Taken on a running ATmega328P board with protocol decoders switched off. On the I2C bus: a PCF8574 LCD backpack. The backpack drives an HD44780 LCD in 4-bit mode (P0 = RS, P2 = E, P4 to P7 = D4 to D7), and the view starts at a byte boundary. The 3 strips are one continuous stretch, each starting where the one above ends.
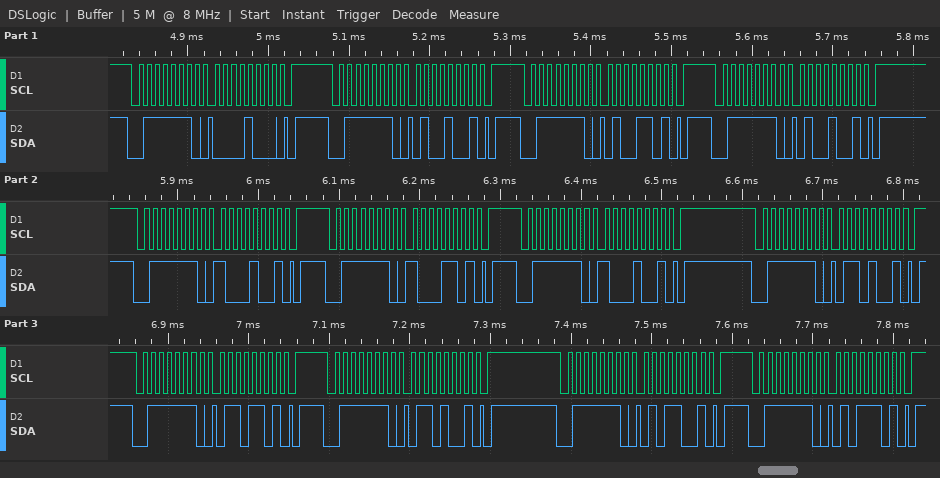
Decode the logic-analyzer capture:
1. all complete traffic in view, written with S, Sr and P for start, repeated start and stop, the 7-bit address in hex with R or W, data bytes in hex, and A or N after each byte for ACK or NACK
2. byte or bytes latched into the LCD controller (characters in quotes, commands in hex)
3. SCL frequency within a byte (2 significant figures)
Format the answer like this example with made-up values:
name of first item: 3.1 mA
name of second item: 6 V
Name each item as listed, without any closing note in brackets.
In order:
all complete traffic in view, written with S, Sr and P for start, repeated start and stop, the 7-bit address in hex with R or W, data bytes in hex, and A or N after each byte for ACK or NACK: S 3FW A 08 A P S 3FW A 49 A P S 3FW A 4D A P S 3FW A 49 A P S 3FW A 89 A P S 3FW A 8D A P S 3FW A 89 A P S 3FW A 69 A P S 3FW A 6D A P S 3FW A 69 A P S 3FW A 59 A P S 3FW A 5D A P
byte or bytes latched into the LCD controller: 'H'
SCL frequency within a byte: 100 kHz
